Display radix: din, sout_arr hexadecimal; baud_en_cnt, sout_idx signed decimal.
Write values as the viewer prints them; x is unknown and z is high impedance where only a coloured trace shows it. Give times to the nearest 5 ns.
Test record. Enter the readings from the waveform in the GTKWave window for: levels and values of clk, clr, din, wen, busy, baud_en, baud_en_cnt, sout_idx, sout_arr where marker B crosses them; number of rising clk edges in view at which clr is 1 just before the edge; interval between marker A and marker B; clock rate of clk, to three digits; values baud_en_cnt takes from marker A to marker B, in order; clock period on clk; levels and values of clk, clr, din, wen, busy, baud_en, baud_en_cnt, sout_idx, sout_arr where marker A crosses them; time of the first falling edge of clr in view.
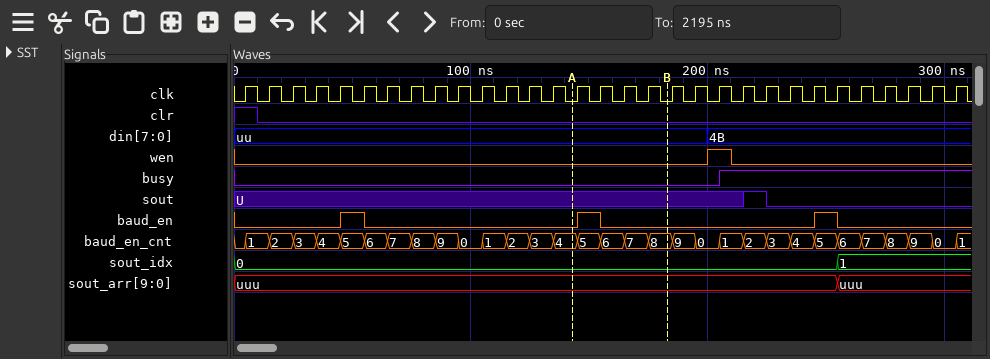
clk=0, clr=0, din=uu, wen=0, busy=0, baud_en=0, baud_en_cnt=8, sout_idx=0, sout_arr=uuu
1
40 ns
100 MHz
4, 5, 6, 7, 8
10 ns
clk=0, clr=0, din=uu, wen=0, busy=0, baud_en=0, baud_en_cnt=4, sout_idx=0, sout_arr=uuu
10 ns
